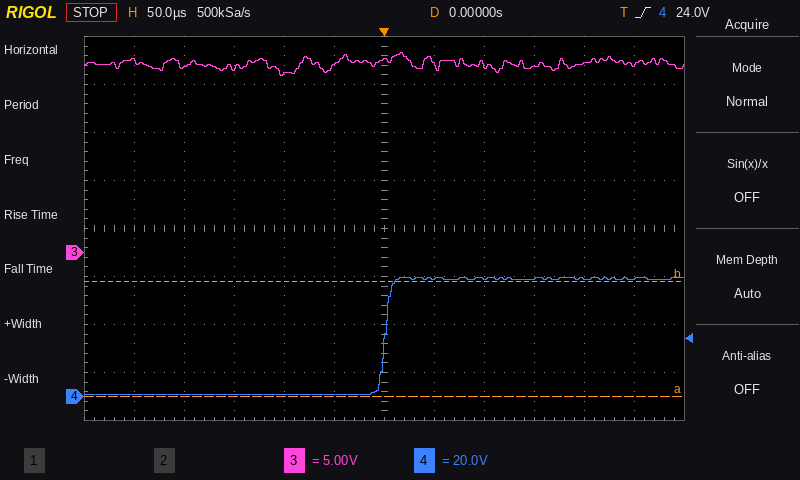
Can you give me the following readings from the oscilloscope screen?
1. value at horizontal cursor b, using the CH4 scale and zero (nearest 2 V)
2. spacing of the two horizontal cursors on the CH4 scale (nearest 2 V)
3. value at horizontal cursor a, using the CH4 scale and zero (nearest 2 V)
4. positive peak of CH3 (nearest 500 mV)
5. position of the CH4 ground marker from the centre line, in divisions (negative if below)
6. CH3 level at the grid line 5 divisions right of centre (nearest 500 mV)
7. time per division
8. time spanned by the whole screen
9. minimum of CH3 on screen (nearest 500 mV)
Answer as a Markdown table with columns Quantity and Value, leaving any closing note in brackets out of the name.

| Quantity | Value |
|---|---|
| value at horizontal cursor b, using the CH4 scale and zero | 48 V |
| spacing of the two horizontal cursors on the CH4 scale | 48 V |
| value at horizontal cursor a, using the CH4 scale and zero | 0 V |
| positive peak of CH3 | 21.0 V |
| position of the CH4 ground marker from the centre line, in divisions | -3.5 div |
| CH3 level at the grid line 5 divisions right of centre | 19.5 V |
| time per division | 50 µs |
| time spanned by the whole screen | 600 µs |
| minimum of CH3 on screen | 18.5 V |
